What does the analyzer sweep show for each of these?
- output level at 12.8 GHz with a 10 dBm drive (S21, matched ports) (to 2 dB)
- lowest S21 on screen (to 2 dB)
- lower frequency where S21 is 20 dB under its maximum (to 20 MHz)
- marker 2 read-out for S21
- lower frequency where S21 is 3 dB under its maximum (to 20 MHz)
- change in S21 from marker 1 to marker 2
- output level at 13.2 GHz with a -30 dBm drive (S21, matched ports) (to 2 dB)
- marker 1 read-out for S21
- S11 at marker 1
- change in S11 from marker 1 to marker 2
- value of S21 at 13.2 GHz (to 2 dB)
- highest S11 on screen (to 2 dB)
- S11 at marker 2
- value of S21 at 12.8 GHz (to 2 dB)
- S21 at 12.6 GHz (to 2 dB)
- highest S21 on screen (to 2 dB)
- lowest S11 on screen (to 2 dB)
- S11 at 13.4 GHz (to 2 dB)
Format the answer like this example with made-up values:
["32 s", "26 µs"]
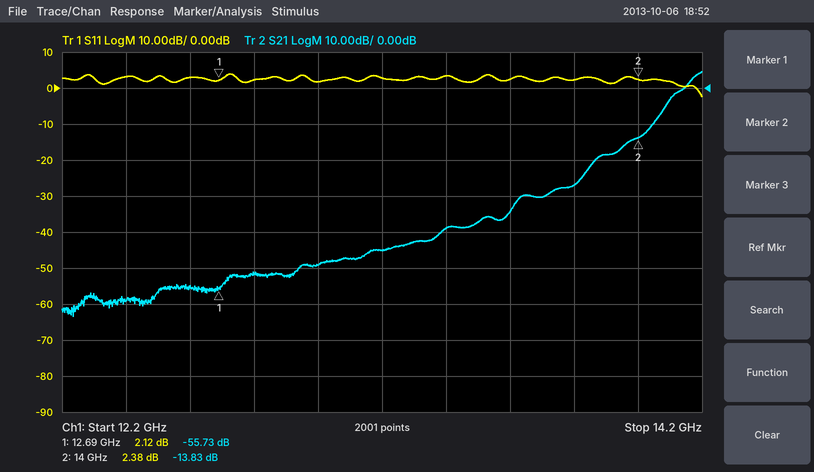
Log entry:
["-42 dBm", "-64 dB", "13.96 GHz", "-13.83 dB", "14.16 GHz", "41.90 dB", "-76 dBm", "-55.73 dB", "2.12 dB", "0.26 dB", "-46 dB", "4 dB", "2.38 dB", "-52 dB", "-56 dB", "4 dB", "-2 dB", "4 dB"]
